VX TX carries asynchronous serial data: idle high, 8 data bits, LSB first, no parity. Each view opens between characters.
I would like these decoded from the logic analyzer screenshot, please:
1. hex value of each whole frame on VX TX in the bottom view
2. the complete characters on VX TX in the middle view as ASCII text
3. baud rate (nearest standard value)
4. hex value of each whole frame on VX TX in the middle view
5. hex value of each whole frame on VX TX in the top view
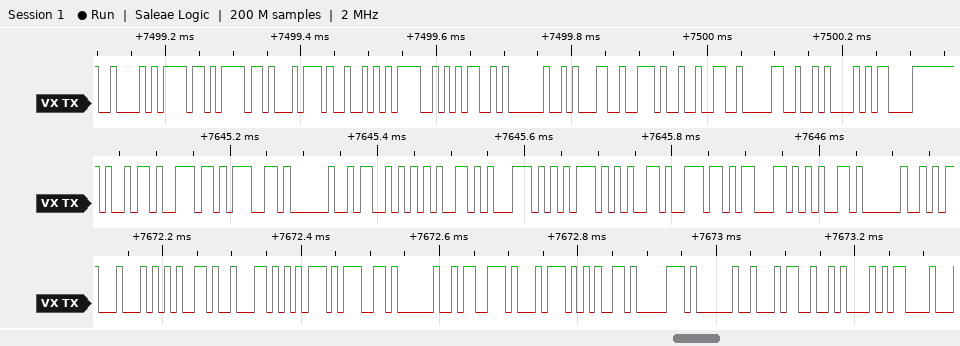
44, 65, 62, 75, 67, 20, 73, 74, 65, 70, 20, 34, 0A, 0D
"ing Sequence "
115200 baud
69, 6E, 67, 20, 53, 65, 71, 75, 65, 6E, 63, 65, 20
42, 6F, 6F, 74, 52, 4F, 4D, 20, 31, 2E, 32, 30, 0A, 0D
